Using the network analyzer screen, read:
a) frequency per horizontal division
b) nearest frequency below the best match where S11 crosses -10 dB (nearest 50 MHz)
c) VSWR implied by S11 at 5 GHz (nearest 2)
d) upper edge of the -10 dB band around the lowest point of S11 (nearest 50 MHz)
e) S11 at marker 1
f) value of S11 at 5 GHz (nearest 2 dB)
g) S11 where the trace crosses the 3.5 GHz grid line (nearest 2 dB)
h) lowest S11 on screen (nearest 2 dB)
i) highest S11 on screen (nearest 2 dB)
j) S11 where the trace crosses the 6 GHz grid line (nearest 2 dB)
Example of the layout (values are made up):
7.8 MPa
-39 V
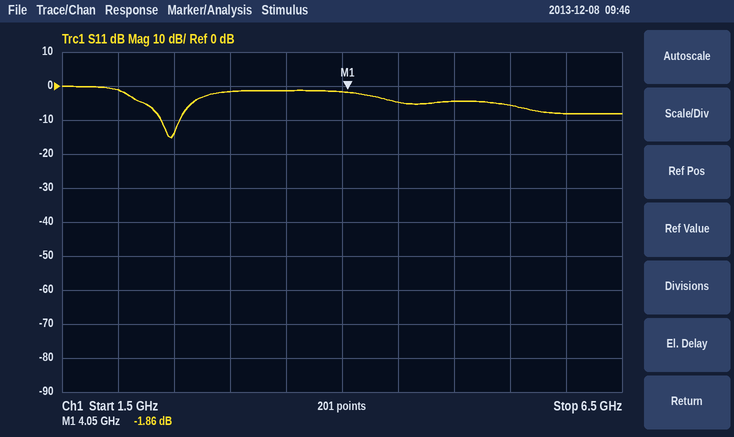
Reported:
500 MHz
2.40 GHz
4
2.55 GHz
-1.86 dB
-4 dB
-2 dB
-16 dB
0 dB
-8 dB
